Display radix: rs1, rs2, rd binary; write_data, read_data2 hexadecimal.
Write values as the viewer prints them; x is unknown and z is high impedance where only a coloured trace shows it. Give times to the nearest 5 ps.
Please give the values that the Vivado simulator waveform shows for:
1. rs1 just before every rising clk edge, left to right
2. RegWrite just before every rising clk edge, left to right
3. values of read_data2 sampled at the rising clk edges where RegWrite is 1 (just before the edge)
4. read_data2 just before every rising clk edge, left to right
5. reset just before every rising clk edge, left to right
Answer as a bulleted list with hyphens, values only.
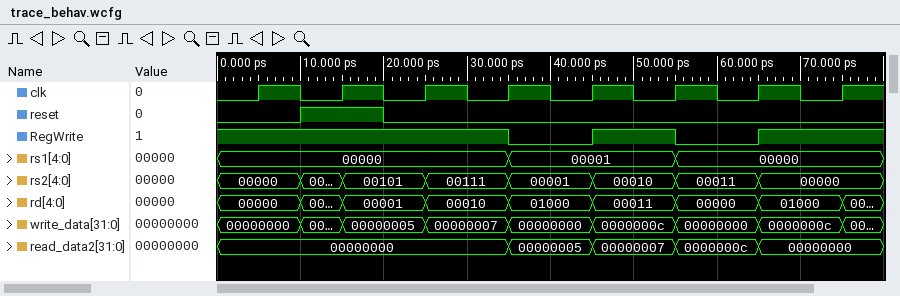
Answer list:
- 00000, 00000, 00000, 00000, 00001, 00001, 00000, 00000
- 1 1 1 1 0 1 0 1
- 00000000, 00000000, 00000000, 00000000, 00000007, 00000000
- 00000000, 00000000, 00000000, 00000000, 00000005, 00000007, 0000000c, 00000000
- 0 1 0 0 0 0 0 0
